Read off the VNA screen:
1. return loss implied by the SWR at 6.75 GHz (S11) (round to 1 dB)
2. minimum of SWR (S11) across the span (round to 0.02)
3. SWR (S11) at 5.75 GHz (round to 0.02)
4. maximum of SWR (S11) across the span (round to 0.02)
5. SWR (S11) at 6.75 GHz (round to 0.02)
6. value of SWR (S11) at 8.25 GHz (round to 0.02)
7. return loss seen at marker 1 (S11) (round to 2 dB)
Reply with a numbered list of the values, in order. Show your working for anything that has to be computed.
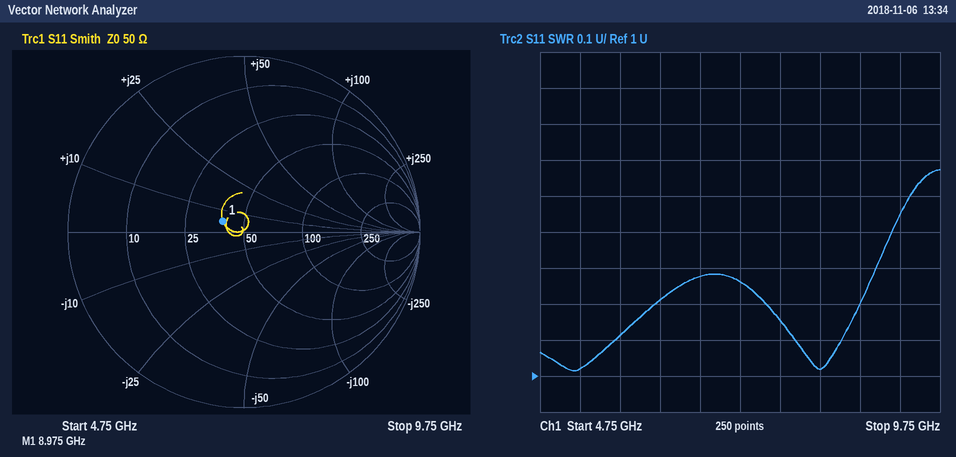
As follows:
1. −20 log10((1.28 − 1)/(1.28 + 1)) ≈ 18 dB
2. 1.02
3. 1.12
4. 1.58
5. 1.28
6. 1.02
7. 18 dB
